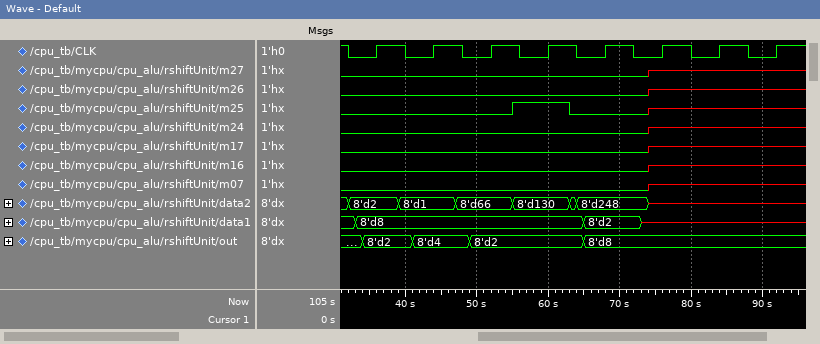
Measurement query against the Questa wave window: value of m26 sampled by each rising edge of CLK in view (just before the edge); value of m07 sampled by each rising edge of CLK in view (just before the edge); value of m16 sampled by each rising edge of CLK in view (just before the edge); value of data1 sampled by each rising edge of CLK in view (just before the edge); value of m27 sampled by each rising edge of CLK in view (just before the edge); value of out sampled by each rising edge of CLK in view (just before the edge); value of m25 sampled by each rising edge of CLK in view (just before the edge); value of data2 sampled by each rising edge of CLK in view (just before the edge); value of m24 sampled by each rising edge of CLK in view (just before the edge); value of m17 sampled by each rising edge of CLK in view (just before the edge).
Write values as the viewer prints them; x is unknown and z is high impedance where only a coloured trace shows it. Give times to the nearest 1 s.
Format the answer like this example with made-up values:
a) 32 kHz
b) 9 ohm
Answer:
a) 0 0 0 0 0 x x x
b) 0 0 0 0 0 x x x
c) 0 0 0 0 0 x x x
d) 8'd8, 8'd8, 8'd8, 8'd8, 8'd2, x, x, x
e) 0 0 0 0 0 x x x
f) 8'd2, 8'd4, 8'd2, 8'd2, 8'd8, 8'd8, 8'd8, 8'd8
g) 0 0 0 1 0 x x x
h) 8'd2, 8'd1, 8'd66, 8'd130, 8'd248, x, x, x
i) 0 0 0 0 0 x x x
j) 0 0 0 0 0 x x x
